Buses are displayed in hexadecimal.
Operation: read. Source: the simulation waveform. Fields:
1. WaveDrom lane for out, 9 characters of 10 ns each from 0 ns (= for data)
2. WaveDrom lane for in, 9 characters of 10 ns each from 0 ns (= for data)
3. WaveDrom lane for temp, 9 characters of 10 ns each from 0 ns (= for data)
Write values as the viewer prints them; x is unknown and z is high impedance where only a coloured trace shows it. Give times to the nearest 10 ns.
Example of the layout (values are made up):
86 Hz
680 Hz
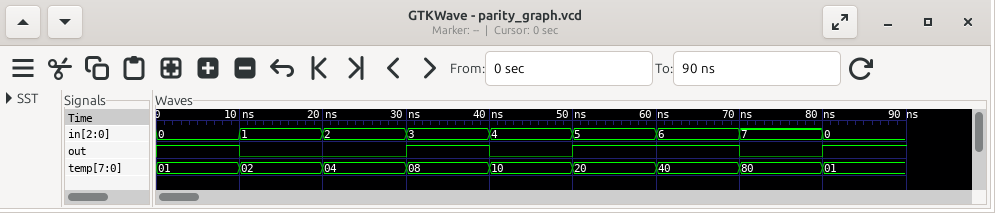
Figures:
{name: 'out', wave: '10.101.01'}
{name: 'in', wave: '=========', data: '0 1 2 3 4 5 6 7 0'}
{name: 'temp', wave: '=========', data: '01 02 04 08 10 20 40 80 01'}
